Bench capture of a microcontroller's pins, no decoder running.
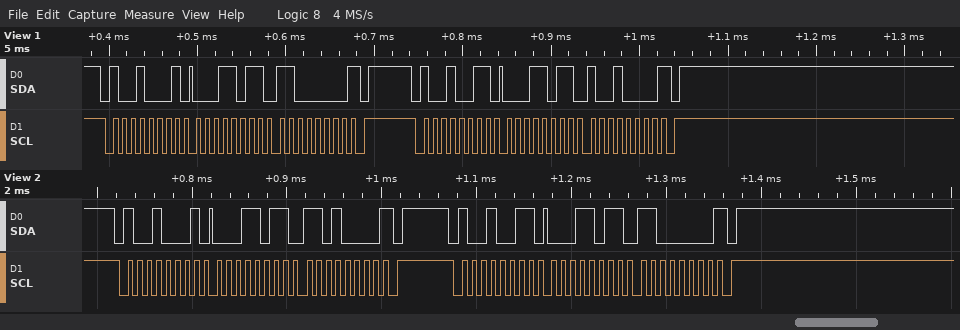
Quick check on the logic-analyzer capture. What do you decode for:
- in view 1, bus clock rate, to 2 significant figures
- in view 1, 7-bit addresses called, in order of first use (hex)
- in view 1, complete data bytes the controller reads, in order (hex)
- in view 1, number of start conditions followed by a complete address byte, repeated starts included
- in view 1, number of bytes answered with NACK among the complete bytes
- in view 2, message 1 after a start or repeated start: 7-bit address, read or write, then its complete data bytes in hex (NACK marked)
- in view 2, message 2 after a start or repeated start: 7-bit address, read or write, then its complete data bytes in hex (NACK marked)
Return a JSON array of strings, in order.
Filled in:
["100 kHz", "0x48 0x49", "1B C0 1B 90", "2", "2", "0x48 read: 1B D0 NACK", "0x49 read: 1B C0 NACK"]
